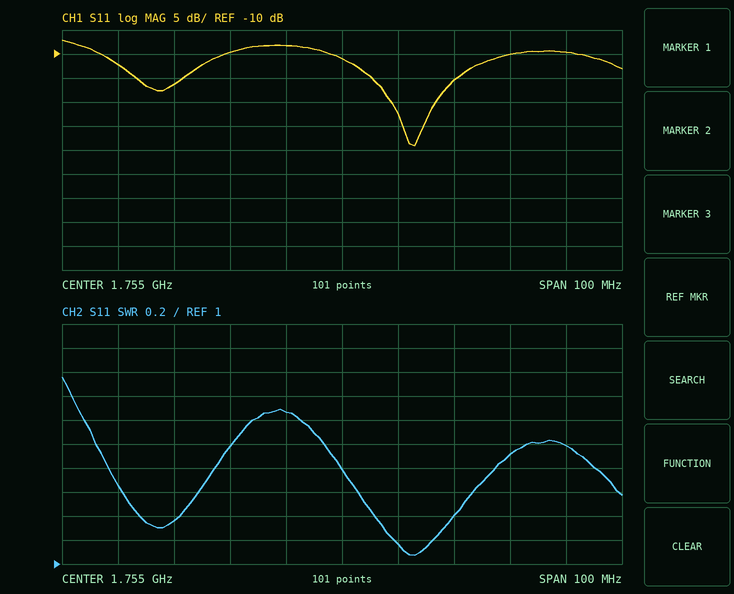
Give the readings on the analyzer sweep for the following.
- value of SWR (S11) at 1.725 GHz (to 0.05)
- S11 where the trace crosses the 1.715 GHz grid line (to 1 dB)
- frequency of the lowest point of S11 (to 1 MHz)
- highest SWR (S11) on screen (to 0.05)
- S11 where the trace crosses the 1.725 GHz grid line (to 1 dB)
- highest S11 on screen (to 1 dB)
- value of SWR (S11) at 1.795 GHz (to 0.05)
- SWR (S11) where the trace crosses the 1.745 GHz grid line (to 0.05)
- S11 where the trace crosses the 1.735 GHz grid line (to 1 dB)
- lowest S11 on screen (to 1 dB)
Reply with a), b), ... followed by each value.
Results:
a) 1.35
b) -12 dB
c) 1.768 GHz
d) 2.55
e) -16 dB
f) -7 dB
g) 2.00
h) 2.25
i) -10 dB
j) -29 dB
